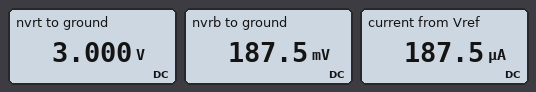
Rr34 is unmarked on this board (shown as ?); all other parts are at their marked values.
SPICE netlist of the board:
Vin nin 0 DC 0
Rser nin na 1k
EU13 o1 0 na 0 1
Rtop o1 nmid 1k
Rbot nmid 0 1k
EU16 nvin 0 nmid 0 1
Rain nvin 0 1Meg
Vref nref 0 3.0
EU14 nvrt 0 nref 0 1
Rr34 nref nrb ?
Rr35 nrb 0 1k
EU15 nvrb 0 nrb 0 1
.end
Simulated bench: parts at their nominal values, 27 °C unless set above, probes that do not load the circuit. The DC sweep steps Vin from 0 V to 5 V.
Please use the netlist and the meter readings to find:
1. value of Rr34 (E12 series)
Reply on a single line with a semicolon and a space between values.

15 kΩ
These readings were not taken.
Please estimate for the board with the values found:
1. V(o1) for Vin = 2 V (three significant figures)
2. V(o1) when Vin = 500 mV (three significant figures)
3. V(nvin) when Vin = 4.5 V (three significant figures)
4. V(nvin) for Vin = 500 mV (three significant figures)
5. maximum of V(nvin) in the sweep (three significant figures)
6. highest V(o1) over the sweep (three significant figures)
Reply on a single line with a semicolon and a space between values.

2.00 V; 500 mV; 2.25 V; 250 mV; 2.50 V; 5.00 V
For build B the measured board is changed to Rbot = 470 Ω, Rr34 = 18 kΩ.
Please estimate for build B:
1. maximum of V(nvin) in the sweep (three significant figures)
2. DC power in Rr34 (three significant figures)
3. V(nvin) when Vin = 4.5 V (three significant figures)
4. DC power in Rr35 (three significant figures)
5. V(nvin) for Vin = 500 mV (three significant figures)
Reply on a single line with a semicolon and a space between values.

1.60 V; 449 µW; 1.44 V; 24.9 µW; 160 mV
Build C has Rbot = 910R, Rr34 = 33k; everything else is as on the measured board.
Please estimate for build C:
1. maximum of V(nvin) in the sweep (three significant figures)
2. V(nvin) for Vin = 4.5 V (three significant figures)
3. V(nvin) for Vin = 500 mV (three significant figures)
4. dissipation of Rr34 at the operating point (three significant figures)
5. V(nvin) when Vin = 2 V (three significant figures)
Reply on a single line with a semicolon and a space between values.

2.38 V; 2.14 V; 238 mV; 257 µW; 953 mV
